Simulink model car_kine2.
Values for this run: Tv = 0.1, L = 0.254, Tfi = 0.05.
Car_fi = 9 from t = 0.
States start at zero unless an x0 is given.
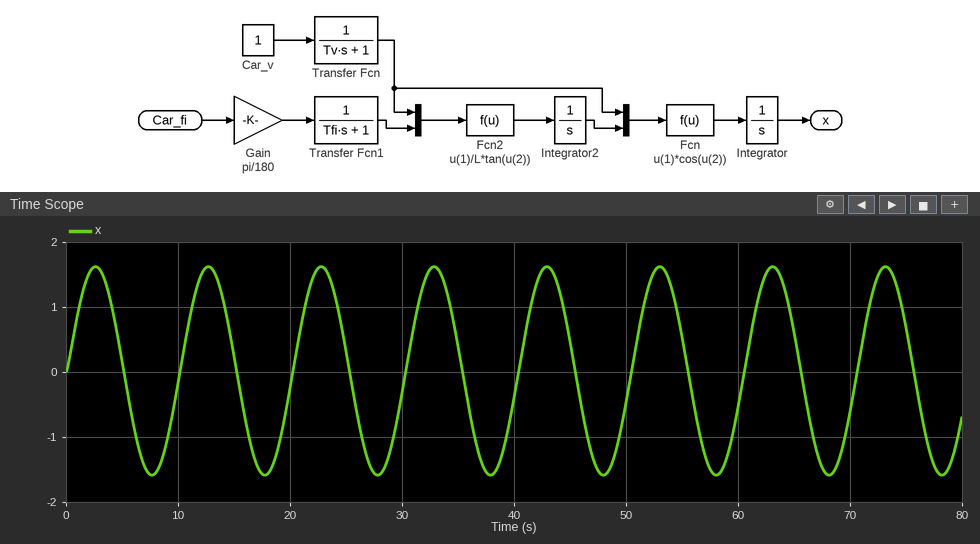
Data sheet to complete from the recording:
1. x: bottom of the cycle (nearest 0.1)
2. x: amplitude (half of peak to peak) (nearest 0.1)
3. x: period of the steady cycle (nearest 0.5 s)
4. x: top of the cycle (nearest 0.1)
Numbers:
-1.6
1.6
10.0 s
1.6
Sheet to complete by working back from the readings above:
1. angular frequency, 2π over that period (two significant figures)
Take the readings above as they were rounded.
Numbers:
0.63 rad/s
